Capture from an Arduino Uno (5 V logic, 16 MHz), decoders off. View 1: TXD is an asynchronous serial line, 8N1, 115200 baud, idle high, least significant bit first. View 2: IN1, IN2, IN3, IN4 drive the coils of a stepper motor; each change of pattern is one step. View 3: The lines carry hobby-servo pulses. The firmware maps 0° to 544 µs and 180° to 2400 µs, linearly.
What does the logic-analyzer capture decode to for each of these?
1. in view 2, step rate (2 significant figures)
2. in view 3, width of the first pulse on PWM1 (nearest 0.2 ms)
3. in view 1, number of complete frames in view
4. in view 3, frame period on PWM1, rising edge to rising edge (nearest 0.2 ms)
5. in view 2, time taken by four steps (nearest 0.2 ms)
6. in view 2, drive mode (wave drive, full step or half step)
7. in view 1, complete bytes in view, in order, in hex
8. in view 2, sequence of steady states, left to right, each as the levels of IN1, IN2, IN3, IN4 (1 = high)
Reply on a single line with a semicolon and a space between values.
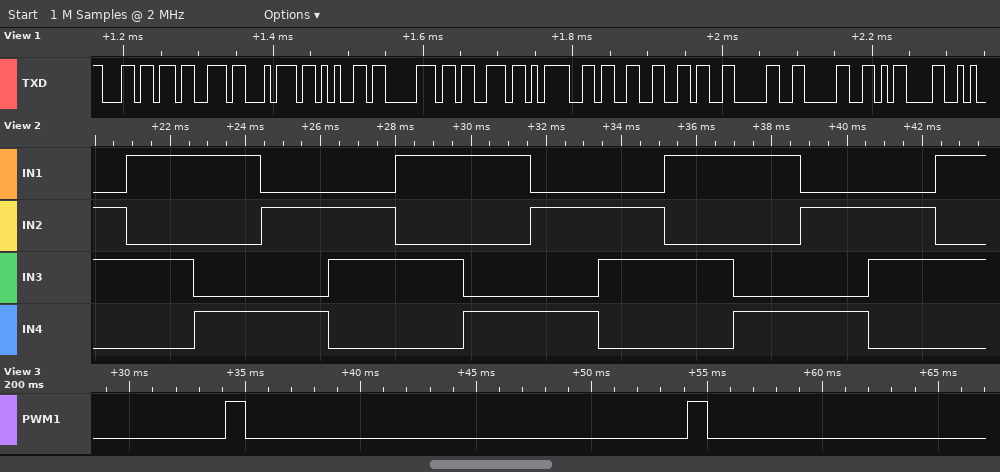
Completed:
560 steps/s; 0.8 ms; 12; 20.0 ms; 7.2 ms; full step; 0x6C 0x73 0x74 0x65 0x70 0x73 0x3D 0x33 0x36 0x30 0x30 0x0D; 0110 1010 1001 0101 0110 1010 1001 0101 0110 1010 1001 0101 0110 1010
